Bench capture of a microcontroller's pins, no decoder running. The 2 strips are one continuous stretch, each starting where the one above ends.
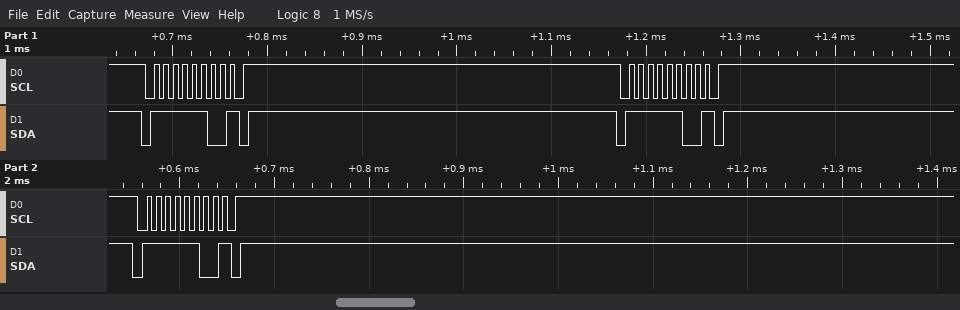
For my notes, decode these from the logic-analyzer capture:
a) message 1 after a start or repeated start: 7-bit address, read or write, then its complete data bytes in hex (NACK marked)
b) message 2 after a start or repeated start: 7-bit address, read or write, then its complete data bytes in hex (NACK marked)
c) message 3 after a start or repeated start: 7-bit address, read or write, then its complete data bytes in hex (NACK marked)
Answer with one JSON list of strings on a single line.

["0x7E write NACK", "0x7E write NACK", "0x7E write NACK"]
